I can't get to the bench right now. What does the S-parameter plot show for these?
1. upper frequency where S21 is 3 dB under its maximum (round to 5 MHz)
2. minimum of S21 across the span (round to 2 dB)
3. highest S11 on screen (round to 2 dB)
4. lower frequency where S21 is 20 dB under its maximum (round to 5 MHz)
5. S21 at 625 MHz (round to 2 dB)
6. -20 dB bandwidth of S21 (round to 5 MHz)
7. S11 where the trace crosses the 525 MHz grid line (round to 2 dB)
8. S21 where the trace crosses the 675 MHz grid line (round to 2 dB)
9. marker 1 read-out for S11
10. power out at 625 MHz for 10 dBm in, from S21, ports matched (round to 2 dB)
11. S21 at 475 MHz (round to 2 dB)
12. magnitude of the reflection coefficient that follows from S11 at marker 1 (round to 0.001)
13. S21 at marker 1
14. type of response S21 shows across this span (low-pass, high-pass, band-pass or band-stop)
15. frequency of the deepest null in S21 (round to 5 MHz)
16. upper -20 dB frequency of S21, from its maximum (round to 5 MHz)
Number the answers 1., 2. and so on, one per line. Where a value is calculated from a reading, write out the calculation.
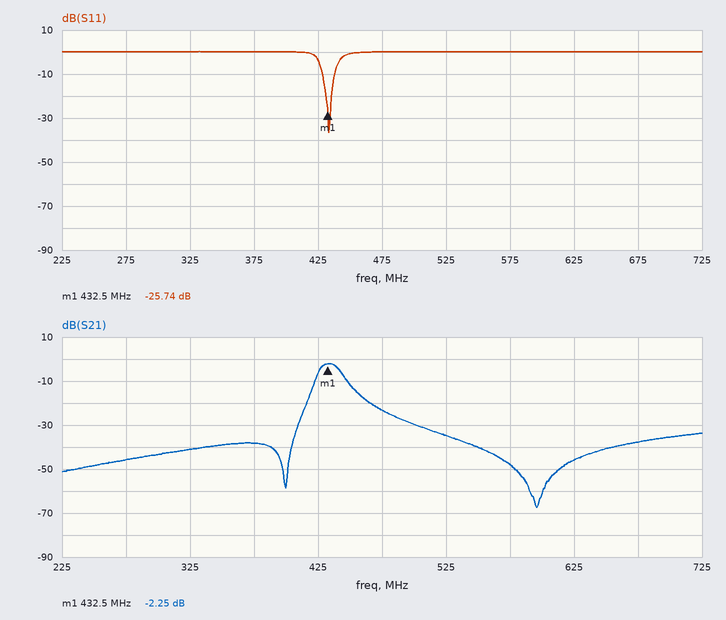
1. 440 MHz
2. -68 dB
3. 0 dB
4. 415 MHz
5. -46 dB
6. 470 MHz − 415 MHz = 55 MHz
7. 0 dB
8. -38 dB
9. -25.74 dB
10. 10 dBm + (-46 dB) = -36 dBm
11. -24 dB
12. 10^(-25.74/20) ≈ 0.052
13. -2.25 dB
14. band-pass
15. 595 MHz
16. 470 MHz
